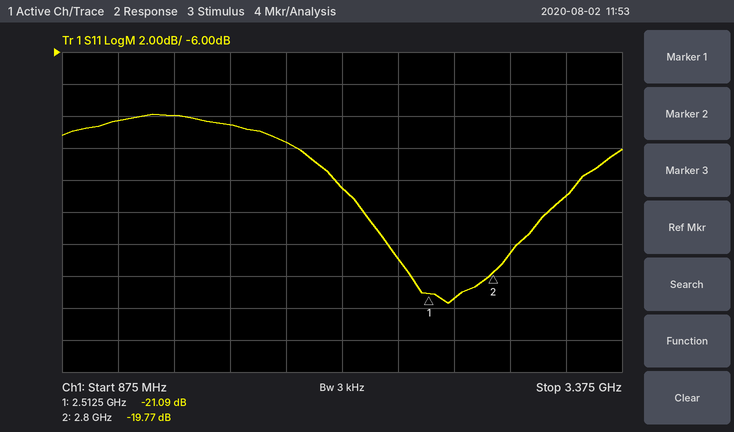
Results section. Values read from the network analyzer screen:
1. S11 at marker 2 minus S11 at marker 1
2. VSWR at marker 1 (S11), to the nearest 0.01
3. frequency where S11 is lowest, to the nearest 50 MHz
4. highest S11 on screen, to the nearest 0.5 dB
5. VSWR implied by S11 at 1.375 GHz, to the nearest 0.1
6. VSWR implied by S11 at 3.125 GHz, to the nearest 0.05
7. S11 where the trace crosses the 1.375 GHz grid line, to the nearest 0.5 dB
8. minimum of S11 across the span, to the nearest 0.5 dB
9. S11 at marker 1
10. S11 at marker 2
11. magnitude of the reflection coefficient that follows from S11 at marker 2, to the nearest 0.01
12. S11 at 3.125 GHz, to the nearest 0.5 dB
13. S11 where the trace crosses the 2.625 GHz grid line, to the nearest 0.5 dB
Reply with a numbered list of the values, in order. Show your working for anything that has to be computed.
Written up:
1. -19.77 − (-21.09) = 1.32 dB
2. (1 + 0.0882)/(1 − 0.0882) ≈ 1.19
3. 2.60 GHz
4. -10.0 dB
5. |Γ| = 10^(-10/20) = 0.3162; VSWR = (1 + 0.3162)/(1 − 0.3162) ≈ 1.9
6. |Γ| = 10^(-15/20) = 0.1778; VSWR = (1 + 0.1778)/(1 − 0.1778) ≈ 1.43, so 1.45 to the nearest 0.05
7. -10.0 dB
8. -21.5 dB
9. -21.09 dB
10. -19.77 dB
11. 10^(-19.77/20) ≈ 0.10
12. -15.0 dB
13. -21.5 dB
